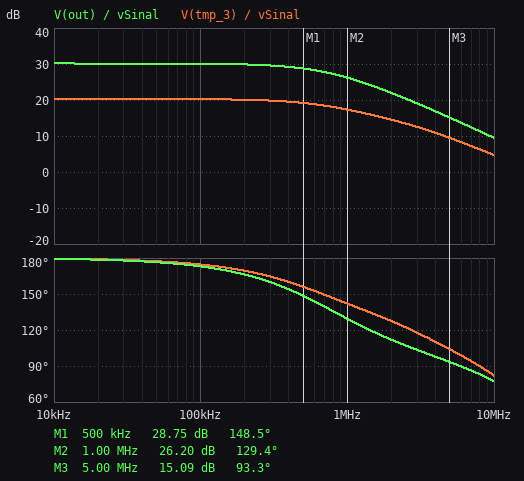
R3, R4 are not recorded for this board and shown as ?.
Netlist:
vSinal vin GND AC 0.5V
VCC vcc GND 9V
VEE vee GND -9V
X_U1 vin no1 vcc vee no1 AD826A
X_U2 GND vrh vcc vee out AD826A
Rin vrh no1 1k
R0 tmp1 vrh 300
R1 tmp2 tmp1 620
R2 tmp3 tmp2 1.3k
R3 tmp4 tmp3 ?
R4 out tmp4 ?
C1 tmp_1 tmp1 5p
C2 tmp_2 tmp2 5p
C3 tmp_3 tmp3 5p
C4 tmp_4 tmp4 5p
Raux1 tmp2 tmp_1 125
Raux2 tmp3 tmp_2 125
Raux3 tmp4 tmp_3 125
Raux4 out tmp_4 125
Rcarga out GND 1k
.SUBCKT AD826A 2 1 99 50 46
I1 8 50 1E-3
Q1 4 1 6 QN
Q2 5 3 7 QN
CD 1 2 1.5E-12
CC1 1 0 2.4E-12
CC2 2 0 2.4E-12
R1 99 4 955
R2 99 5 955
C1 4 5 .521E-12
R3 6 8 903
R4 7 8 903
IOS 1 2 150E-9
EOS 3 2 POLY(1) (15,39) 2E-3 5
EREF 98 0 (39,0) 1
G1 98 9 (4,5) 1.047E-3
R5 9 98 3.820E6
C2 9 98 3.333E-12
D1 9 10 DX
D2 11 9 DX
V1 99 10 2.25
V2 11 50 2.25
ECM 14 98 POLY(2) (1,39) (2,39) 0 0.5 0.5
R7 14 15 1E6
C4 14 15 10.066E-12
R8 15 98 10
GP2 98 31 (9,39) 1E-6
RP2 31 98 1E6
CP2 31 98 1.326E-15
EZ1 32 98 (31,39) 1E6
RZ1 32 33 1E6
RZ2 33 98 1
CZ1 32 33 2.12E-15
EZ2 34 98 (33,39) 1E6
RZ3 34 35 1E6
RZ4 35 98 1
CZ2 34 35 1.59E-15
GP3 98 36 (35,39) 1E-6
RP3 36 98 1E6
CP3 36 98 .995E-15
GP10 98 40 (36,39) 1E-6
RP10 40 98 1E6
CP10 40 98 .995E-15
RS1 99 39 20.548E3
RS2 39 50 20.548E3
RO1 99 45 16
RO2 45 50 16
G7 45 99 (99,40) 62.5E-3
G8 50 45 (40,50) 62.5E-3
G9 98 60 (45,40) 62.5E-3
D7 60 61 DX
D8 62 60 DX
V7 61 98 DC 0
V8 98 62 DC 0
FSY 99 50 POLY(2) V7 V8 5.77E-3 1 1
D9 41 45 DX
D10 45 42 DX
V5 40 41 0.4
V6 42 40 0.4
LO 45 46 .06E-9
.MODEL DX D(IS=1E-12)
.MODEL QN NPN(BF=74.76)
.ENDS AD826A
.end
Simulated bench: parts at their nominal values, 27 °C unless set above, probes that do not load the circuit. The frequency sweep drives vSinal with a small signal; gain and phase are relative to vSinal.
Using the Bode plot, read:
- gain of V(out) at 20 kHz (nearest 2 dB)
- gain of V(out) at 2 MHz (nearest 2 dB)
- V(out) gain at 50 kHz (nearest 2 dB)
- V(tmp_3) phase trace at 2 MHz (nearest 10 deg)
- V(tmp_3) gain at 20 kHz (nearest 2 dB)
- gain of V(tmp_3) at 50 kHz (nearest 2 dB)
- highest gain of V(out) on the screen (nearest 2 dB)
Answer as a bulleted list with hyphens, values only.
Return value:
- 30 dB
- 22 dB
- 30 dB
- 130 deg
- 20 dB
- 20 dB
- 30 dB
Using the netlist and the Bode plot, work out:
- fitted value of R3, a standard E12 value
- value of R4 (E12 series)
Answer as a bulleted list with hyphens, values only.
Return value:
- 8.2 kΩ
- 22 kΩ
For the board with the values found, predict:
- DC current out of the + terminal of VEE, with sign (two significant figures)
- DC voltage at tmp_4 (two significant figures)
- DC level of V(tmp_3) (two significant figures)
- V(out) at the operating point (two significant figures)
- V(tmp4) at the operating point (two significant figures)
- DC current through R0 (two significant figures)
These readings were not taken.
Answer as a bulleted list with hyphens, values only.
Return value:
- -14 mA
- 220 mV
- 72 mV
- 220 mV
- 72 mV
- 6.7 µA
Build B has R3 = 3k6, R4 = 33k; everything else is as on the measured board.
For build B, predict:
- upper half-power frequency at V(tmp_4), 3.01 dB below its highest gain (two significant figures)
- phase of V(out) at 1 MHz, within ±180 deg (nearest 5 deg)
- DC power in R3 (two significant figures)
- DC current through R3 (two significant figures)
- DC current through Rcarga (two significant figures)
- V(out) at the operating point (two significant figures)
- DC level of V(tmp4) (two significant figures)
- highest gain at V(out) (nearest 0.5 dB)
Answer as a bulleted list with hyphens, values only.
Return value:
- 580 kHz
- 120 deg
- 160 nW
- 6.7 µA
- 260 µA
- 260 mV
- 41 mV
- 31.5 dB
